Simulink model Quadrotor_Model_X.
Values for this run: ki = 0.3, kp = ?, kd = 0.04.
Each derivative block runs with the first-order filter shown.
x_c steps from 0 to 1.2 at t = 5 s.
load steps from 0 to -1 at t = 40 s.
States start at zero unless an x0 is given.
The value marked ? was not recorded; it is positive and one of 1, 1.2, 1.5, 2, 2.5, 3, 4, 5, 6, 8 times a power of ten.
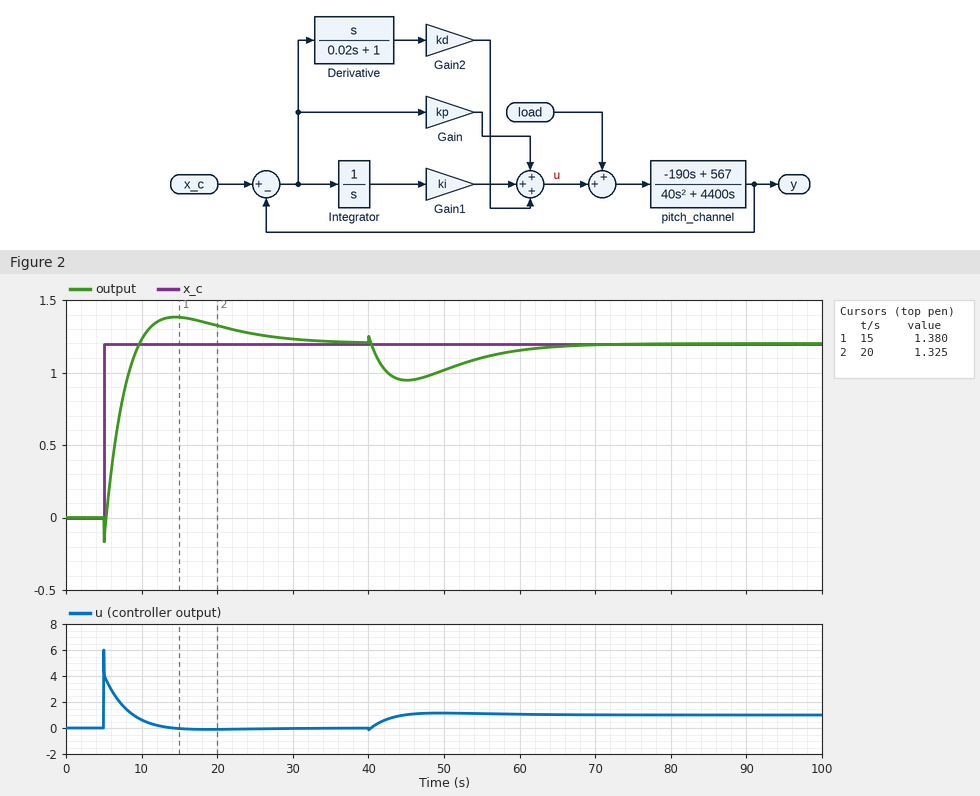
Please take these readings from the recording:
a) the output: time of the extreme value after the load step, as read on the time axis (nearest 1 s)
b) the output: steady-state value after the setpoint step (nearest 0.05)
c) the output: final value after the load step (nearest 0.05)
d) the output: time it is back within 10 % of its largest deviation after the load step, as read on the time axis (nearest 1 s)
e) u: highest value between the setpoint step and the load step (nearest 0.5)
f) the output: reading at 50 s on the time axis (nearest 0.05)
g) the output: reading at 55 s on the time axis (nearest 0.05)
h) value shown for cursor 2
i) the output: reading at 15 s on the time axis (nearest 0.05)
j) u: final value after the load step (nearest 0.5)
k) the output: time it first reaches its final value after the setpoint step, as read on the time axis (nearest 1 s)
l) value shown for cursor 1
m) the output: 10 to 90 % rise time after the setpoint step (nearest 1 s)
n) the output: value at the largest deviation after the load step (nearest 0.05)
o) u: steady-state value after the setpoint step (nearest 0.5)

45 s
1.20
1.20
64 s
6.0
1.00
1.10
1.325
1.40
1.0
10 s
1.380
3 s
0.95
0.0
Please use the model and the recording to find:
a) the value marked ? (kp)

3
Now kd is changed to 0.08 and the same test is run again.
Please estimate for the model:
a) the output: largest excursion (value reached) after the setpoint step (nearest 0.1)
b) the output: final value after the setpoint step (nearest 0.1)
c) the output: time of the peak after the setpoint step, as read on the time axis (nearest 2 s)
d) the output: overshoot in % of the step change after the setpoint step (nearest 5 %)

1.4
1.2
14 s
15 %
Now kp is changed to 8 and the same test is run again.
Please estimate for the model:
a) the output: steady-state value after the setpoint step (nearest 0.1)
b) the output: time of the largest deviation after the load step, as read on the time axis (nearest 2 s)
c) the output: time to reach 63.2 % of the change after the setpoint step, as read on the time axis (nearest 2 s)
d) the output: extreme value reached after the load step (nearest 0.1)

1.2
42 s
6 s
1.1
